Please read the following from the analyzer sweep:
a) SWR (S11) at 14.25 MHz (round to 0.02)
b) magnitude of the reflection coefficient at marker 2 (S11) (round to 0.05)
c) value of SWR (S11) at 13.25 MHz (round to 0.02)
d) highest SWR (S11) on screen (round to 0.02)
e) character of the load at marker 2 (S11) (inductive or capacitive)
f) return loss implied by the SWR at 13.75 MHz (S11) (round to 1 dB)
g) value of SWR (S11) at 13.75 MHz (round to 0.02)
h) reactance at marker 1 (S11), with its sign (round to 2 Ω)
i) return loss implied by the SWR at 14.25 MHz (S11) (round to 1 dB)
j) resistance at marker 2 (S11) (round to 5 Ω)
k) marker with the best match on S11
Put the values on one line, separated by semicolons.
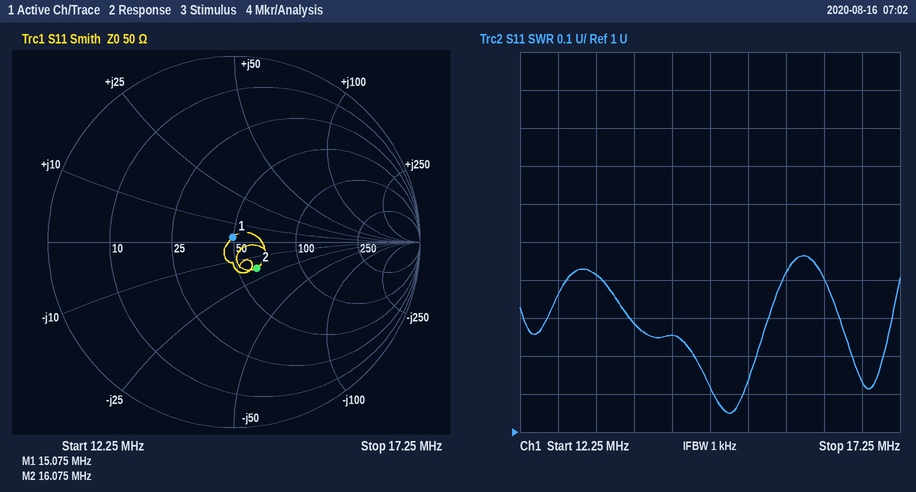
1.26; 0.20; 1.42; 1.46; capacitive; 18 dB; 1.28; +2 Ω; 19 dB; 60 Ω; marker 1
